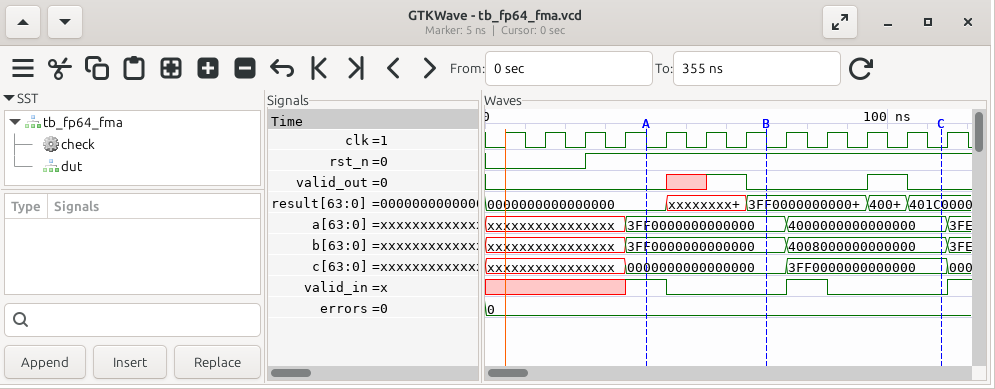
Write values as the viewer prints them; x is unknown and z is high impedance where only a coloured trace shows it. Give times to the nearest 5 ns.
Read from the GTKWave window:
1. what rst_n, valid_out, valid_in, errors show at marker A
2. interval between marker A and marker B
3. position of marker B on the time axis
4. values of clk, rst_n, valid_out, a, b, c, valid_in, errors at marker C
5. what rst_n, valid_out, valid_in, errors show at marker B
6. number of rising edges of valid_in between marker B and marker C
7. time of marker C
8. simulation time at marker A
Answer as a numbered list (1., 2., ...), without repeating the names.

1. rst_n=1, valid_out=0, valid_in=1, errors=0
2. 30 ns
3. 70 ns
4. clk=0, rst_n=1, valid_out=0, a=4000000000000000, b=4008000000000000, c=3FF0000000000000, valid_in=0, errors=0
5. rst_n=1, valid_out=0, valid_in=0, errors=0
6. 1
7. 115 ns
8. 40 ns
